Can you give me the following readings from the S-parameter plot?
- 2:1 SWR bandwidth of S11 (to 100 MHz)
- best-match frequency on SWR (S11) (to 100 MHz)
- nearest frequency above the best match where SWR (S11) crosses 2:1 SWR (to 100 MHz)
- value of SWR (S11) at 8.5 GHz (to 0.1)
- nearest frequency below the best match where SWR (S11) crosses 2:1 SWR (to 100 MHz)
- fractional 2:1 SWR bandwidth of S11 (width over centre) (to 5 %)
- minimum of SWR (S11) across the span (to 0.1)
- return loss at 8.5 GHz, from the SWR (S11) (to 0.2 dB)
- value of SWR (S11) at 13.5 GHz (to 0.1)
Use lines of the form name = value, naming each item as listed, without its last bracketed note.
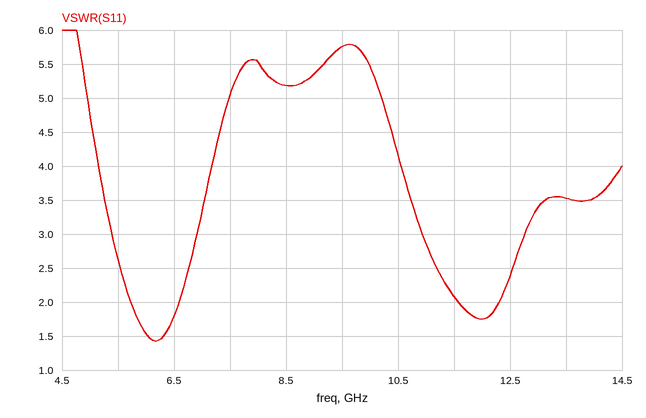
2:1 SWR bandwidth of S11 = 900 MHz
best-match frequency on SWR (S11) = 6.2 GHz
nearest frequency above the best match where SWR (S11) crosses 2:1 SWR = 6.6 GHz
value of SWR (S11) at 8.5 GHz = 5.2
nearest frequency below the best match where SWR (S11) crosses 2:1 SWR = 5.7 GHz
fractional 2:1 SWR bandwidth of S11 (width over centre) = 15 %
minimum of SWR (S11) across the span = 1.4
return loss at 8.5 GHz, from the SWR (S11) = 3.4 dB
value of SWR (S11) at 13.5 GHz = 3.5
